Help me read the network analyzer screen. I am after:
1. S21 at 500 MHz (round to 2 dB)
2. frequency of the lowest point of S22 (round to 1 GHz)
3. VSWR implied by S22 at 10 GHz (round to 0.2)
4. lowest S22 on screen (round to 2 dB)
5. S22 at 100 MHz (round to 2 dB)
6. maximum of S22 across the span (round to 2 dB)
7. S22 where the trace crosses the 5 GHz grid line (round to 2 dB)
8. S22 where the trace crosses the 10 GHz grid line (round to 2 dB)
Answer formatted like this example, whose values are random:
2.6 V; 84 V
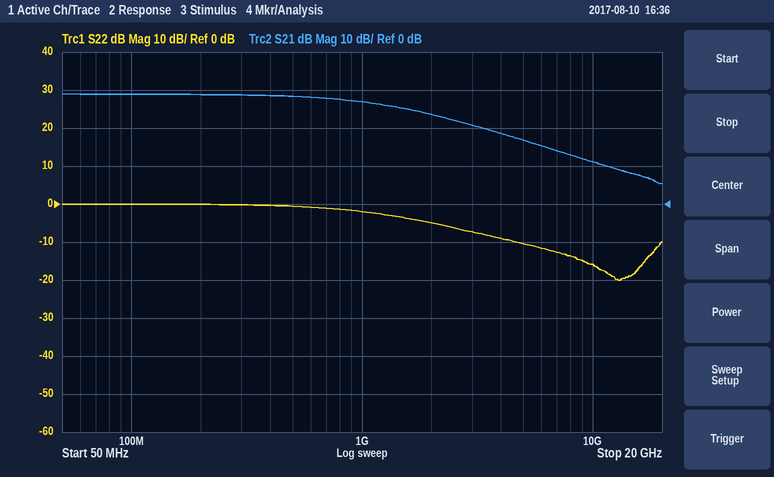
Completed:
28 dB; 13 GHz; 1.4; -20 dB; 0 dB; 0 dB; -10 dB; -16 dB
